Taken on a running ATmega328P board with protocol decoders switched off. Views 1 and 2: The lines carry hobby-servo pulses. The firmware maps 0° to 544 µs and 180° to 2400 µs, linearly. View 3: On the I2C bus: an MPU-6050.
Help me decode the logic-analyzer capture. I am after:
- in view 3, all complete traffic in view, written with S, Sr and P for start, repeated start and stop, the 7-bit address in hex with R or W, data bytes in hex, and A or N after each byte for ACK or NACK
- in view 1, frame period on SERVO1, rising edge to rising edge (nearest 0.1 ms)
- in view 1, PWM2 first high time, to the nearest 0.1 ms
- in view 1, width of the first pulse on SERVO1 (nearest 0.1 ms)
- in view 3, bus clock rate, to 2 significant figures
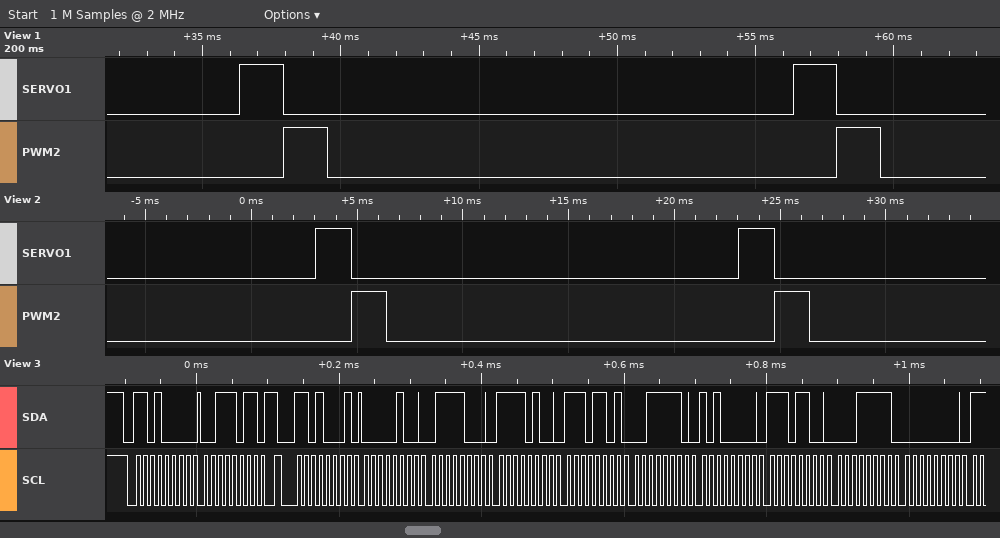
S 68W A 3B A Sr 68R A 04 A 78 A F4 A ED A 3E A A0 A EC A 1F A 00 A
20.0 ms
1.6 ms
1.6 ms
100 kHz
